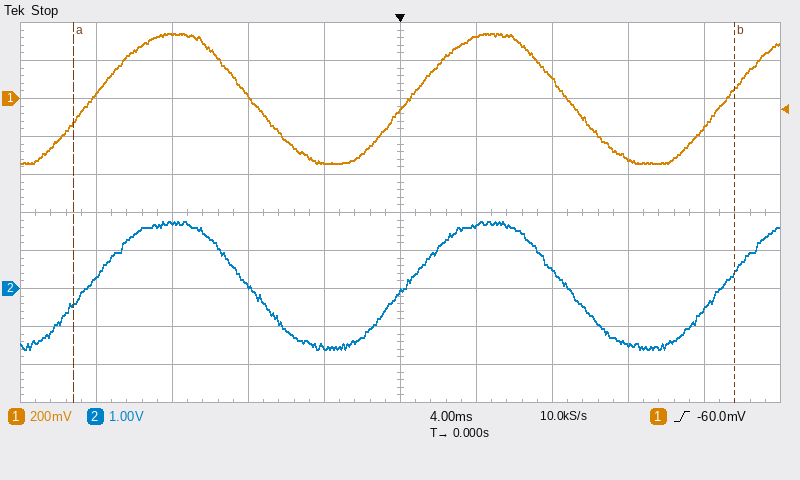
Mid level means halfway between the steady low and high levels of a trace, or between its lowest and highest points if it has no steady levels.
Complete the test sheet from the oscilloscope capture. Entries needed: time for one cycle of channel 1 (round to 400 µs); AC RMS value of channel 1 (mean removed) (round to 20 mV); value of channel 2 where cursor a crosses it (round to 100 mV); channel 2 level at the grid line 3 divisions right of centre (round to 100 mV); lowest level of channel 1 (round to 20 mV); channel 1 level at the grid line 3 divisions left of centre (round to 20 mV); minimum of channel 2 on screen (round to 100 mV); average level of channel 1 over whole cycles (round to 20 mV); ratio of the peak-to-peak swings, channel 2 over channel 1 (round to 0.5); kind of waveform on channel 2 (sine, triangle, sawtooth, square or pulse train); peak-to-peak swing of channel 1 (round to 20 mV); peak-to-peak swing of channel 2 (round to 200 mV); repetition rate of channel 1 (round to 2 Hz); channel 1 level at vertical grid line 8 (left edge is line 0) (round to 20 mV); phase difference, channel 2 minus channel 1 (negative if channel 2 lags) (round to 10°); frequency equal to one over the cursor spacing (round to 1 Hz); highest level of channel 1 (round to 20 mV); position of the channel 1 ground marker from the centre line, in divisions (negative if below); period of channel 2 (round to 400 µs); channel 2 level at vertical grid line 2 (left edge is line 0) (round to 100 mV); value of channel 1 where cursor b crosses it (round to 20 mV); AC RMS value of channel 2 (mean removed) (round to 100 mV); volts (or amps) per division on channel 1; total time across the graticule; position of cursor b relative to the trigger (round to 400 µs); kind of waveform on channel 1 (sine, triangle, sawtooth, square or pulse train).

16.8 ms
240 mV
-400 mV
-1.5 V
-340 mV
340 mV
-1.6 V
0 mV
5.0
sine
680 mV
3.4 V
60 Hz
-320 mV
0°
29 Hz
340 mV
+3.0 div
16.8 ms
1.7 V
60 mV
1.2 V
200 mV
40 ms
+17.6 ms
sine
